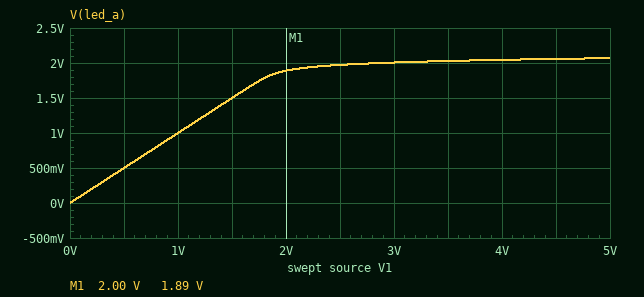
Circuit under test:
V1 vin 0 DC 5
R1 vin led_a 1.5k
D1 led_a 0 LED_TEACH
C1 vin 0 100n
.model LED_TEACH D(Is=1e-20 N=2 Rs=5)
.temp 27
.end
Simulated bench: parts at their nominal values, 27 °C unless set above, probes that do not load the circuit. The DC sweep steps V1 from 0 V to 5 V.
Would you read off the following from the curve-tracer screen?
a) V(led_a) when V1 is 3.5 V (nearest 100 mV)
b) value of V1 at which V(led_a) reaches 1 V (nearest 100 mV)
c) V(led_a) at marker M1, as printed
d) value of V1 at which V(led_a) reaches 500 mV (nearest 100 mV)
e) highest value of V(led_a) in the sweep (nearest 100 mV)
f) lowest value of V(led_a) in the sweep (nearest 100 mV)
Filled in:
2.0 V
1.0 V
1.89 V
500 mV
2.1 V
0 V
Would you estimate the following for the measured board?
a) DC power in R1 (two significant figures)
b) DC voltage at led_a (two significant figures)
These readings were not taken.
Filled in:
5.7 mW
2.1 V
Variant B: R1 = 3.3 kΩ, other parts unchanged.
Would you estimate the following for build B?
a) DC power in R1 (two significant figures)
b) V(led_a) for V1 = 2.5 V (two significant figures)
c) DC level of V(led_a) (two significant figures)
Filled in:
2.7 mW
1.9 V
2.0 V
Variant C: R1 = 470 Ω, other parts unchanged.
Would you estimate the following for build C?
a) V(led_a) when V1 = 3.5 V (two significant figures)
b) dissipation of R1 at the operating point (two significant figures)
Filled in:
2.1 V
17 mW
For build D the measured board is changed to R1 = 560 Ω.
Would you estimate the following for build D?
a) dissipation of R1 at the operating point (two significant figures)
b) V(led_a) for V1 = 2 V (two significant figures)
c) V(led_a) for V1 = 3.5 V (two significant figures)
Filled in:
15 mW
1.9 V
2.1 V
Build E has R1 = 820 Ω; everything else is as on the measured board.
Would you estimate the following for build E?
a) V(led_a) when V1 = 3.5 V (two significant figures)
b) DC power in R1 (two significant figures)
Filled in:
2.1 V
10 mW
